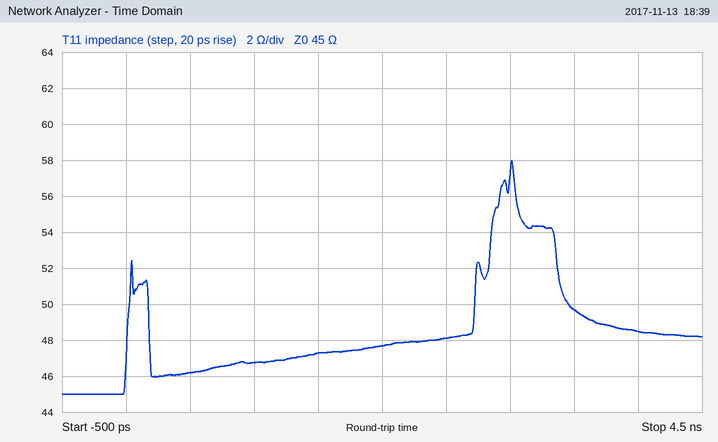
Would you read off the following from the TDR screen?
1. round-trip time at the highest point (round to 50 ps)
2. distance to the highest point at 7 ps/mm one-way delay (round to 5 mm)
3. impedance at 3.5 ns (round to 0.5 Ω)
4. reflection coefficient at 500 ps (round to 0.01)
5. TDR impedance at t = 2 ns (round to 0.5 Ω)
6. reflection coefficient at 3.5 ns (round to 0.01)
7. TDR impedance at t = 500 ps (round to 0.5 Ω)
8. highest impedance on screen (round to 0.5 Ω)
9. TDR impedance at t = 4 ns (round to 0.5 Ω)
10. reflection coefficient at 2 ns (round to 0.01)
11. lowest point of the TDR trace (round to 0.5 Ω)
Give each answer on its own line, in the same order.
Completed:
3.00 ns
215 mm
49.5 Ω
+0.01
47.5 Ω
+0.05
46.0 Ω
58.0 Ω
48.5 Ω
+0.03
45.0 Ω
